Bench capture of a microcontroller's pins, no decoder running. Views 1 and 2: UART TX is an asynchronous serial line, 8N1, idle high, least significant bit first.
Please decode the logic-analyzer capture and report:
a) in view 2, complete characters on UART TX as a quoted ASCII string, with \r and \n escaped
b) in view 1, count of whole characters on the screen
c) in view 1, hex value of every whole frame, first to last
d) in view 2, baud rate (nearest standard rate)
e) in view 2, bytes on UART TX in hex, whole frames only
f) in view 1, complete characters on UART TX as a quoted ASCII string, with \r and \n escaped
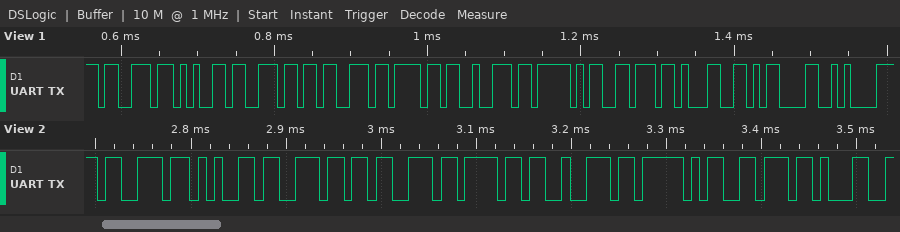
"sensor_v1"
11
73 65 6E 73 6F 72 5F 76 31 0D 0A
115200 baud
0x73 0x65 0x6E 0x73 0x6F 0x72 0x5F 0x76 0x31
"sensor_v1\r\n"
